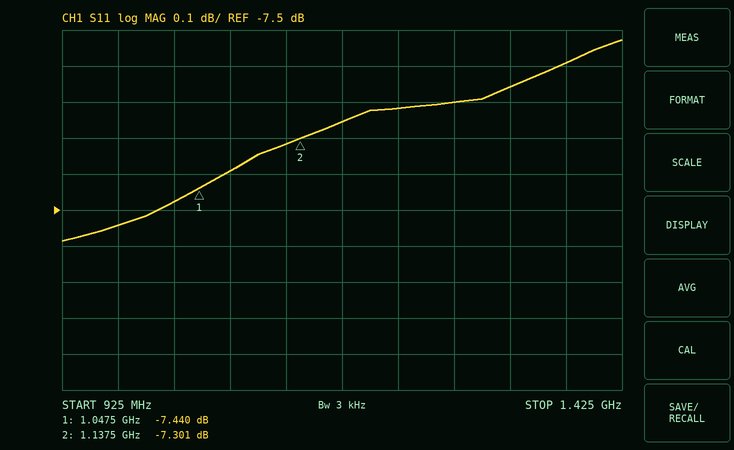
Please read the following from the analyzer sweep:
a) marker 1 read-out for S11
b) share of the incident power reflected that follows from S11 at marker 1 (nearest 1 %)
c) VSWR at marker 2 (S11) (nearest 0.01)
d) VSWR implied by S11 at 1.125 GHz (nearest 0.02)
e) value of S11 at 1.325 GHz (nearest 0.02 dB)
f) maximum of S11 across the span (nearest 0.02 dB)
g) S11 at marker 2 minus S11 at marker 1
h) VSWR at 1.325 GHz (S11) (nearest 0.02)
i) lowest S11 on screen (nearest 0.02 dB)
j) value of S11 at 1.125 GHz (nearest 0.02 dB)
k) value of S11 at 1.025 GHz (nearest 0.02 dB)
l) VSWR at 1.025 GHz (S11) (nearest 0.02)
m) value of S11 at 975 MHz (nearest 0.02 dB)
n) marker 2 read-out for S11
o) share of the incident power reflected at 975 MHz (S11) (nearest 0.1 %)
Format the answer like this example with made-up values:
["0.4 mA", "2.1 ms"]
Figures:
["-7.440 dB", "18 %", "2.52", "2.52", "-7.16 dB", "-7.02 dB", "0.139 dB", "2.56", "-7.58 dB", "-7.32 dB", "-7.48 dB", "2.46", "-7.54 dB", "-7.301 dB", "17.6 %"]
